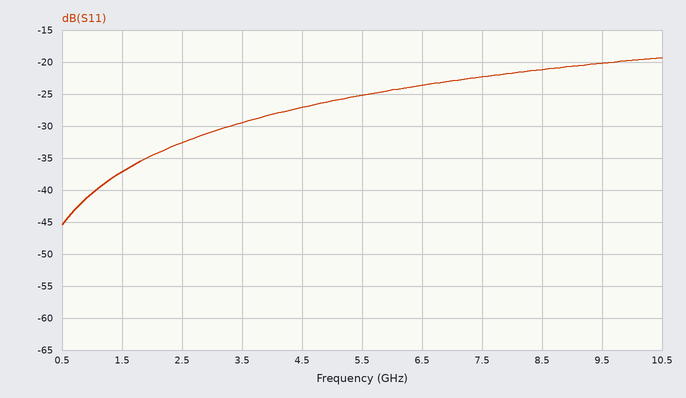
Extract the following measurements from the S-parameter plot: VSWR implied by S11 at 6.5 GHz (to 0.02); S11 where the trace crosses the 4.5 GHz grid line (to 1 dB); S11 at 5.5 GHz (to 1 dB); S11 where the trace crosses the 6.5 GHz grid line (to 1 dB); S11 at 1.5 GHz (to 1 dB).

1.14
-27 dB
-25 dB
-24 dB
-37 dB
